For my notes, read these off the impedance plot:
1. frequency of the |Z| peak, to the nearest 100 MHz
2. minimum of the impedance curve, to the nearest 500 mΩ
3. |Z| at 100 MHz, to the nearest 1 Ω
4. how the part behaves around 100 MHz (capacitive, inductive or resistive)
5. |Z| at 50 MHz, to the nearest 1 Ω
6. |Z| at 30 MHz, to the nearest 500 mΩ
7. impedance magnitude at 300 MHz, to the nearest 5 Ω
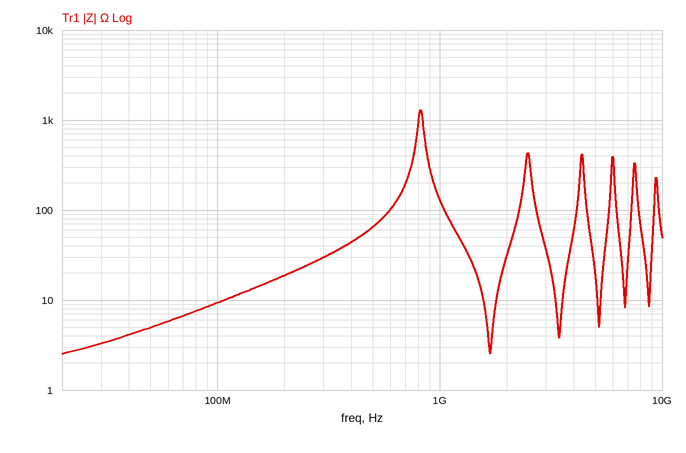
800 MHz
2.5 Ω
9 Ω
inductive
5 Ω
3.5 Ω
30 Ω
